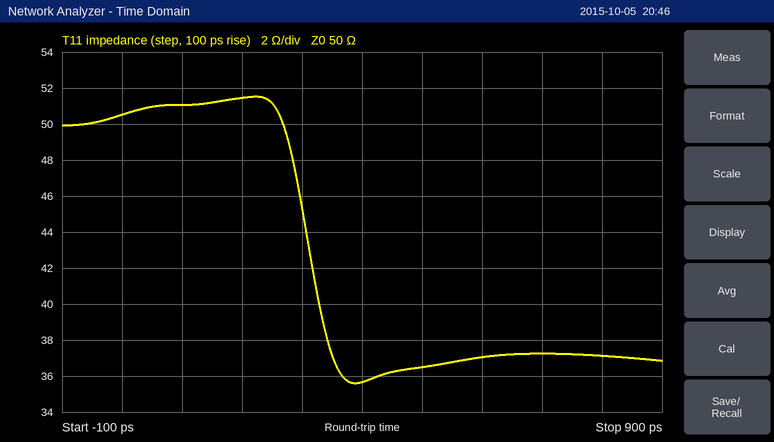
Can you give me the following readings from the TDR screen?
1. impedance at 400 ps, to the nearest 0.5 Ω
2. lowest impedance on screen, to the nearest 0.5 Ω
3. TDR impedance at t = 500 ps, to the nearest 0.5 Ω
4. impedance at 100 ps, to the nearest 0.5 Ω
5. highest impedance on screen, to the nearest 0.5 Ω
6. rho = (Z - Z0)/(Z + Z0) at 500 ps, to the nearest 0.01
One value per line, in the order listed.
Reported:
35.5 Ω
35.5 Ω
36.5 Ω
51.0 Ω
51.5 Ω
-0.16
